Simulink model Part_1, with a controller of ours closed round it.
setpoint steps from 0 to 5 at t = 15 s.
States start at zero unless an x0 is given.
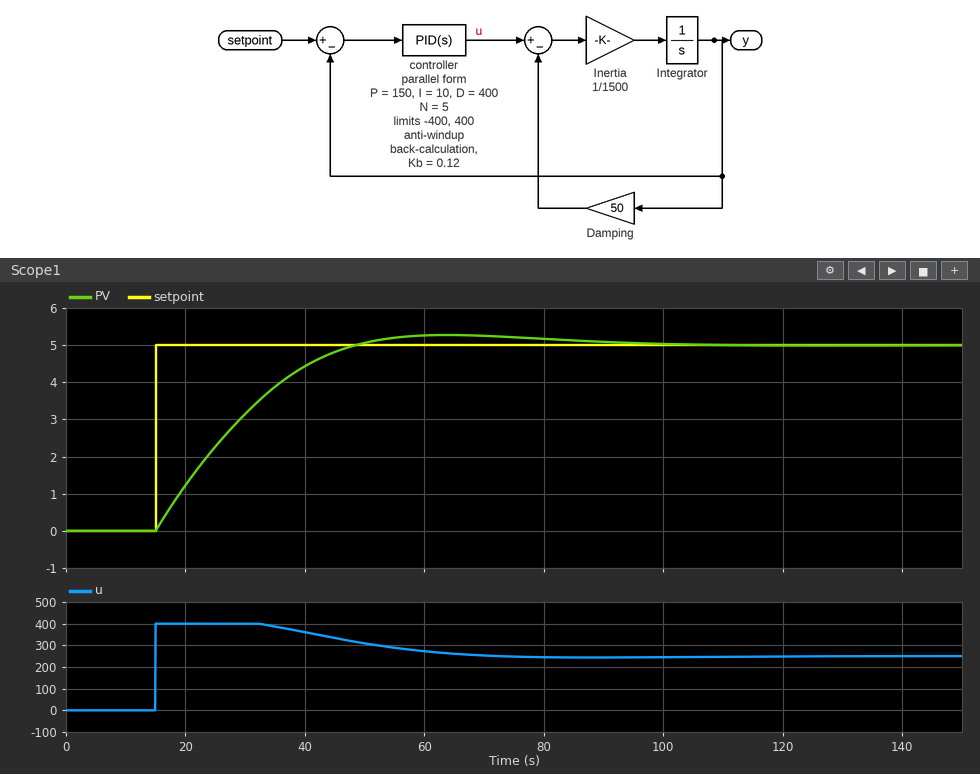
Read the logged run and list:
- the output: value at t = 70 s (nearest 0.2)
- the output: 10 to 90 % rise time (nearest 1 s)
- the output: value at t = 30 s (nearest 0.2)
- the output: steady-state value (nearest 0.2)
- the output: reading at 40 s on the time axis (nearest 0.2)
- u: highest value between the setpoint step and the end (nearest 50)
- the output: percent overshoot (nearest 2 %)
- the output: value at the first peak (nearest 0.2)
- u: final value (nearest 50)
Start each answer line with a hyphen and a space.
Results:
- 5.2
- 24 s
- 3.2
- 5.0
- 4.4
- 400
- 6 %
- 5.2
- 250
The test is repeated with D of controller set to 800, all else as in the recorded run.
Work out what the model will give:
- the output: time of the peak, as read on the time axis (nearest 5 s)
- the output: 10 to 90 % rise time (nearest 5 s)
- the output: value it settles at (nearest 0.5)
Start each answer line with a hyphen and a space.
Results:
- 70 s
- 30 s
- 5.0
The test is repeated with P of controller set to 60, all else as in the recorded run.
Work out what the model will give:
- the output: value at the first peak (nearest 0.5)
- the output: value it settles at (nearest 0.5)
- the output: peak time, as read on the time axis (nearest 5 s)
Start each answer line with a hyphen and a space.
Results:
- 6.0
- 5.0
- 65 s
